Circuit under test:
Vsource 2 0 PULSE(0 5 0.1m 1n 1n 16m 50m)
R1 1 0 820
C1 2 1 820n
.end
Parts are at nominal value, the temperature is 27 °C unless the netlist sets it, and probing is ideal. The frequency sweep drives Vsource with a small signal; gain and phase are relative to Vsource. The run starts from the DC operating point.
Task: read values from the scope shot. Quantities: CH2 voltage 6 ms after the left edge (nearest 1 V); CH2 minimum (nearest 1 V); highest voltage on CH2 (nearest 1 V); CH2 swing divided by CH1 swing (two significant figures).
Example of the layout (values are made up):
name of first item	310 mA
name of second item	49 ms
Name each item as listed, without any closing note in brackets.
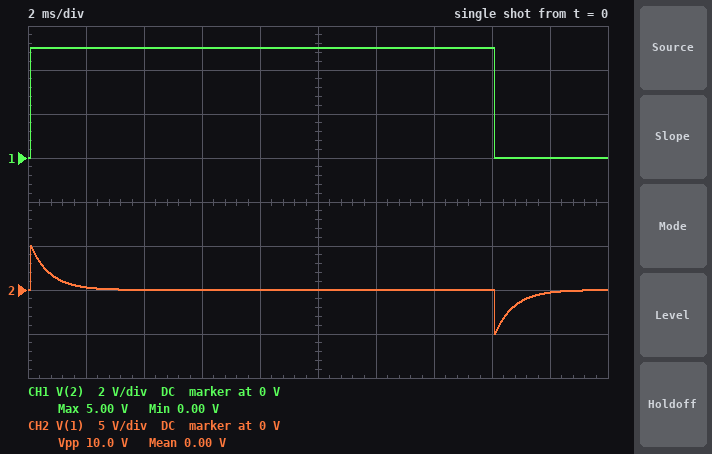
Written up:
CH2 voltage 6 ms after the left edge	0 V
CH2 minimum	-5 V
highest voltage on CH2	5 V
CH2 swing divided by CH1 swing	2.0
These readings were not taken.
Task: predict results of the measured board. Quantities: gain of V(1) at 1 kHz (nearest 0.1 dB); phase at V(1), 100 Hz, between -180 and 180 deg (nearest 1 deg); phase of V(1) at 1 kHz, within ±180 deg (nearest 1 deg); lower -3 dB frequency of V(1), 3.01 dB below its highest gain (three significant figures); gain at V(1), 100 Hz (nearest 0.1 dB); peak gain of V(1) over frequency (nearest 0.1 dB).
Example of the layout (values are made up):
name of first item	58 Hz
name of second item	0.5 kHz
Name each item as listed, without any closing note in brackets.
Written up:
gain of V(1) at 1 kHz	-0.2 dB
phase at V(1), 100 Hz, between -180 and 180 deg	67 deg
phase of V(1) at 1 kHz, within ±180 deg	13 deg
lower -3 dB frequency of V(1), 3.01 dB below its highest gain	237 Hz
gain at V(1), 100 Hz	-8.2 dB
peak gain of V(1) over frequency	0 dB
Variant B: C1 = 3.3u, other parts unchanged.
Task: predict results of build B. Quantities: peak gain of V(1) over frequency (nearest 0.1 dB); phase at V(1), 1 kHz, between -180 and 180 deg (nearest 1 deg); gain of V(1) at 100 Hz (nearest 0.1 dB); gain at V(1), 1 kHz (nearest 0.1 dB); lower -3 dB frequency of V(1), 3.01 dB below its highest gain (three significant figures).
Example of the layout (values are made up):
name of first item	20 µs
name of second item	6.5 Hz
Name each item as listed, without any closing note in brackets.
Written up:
peak gain of V(1) over frequency	0 dB
phase at V(1), 1 kHz, between -180 and 180 deg	3 deg
gain of V(1) at 100 Hz	-1.3 dB
gain at V(1), 1 kHz	0 dB
lower -3 dB frequency of V(1), 3.01 dB below its highest gain	58.8 Hz
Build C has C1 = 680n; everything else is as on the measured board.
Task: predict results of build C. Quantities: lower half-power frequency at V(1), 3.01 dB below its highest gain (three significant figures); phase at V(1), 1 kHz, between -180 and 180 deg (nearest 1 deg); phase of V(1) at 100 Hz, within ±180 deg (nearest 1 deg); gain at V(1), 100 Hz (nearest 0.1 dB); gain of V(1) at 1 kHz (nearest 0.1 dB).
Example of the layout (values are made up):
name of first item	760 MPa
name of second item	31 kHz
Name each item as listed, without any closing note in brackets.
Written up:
lower half-power frequency at V(1), 3.01 dB below its highest gain	285 Hz
phase at V(1), 1 kHz, between -180 and 180 deg	16 deg
phase of V(1) at 100 Hz, within ±180 deg	71 deg
gain at V(1), 100 Hz	-9.6 dB
gain of V(1) at 1 kHz	-0.3 dB
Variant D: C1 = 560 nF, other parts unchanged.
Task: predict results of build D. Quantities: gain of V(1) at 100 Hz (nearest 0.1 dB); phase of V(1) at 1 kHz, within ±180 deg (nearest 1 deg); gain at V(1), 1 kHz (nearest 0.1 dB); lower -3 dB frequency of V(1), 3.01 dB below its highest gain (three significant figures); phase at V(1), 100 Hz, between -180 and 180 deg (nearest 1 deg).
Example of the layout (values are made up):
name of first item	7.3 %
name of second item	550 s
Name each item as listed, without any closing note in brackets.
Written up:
gain of V(1) at 100 Hz	-11.1 dB
phase of V(1) at 1 kHz, within ±180 deg	19 deg
gain at V(1), 1 kHz	-0.5 dB
lower -3 dB frequency of V(1), 3.01 dB below its highest gain	347 Hz
phase at V(1), 100 Hz, between -180 and 180 deg	74 deg
